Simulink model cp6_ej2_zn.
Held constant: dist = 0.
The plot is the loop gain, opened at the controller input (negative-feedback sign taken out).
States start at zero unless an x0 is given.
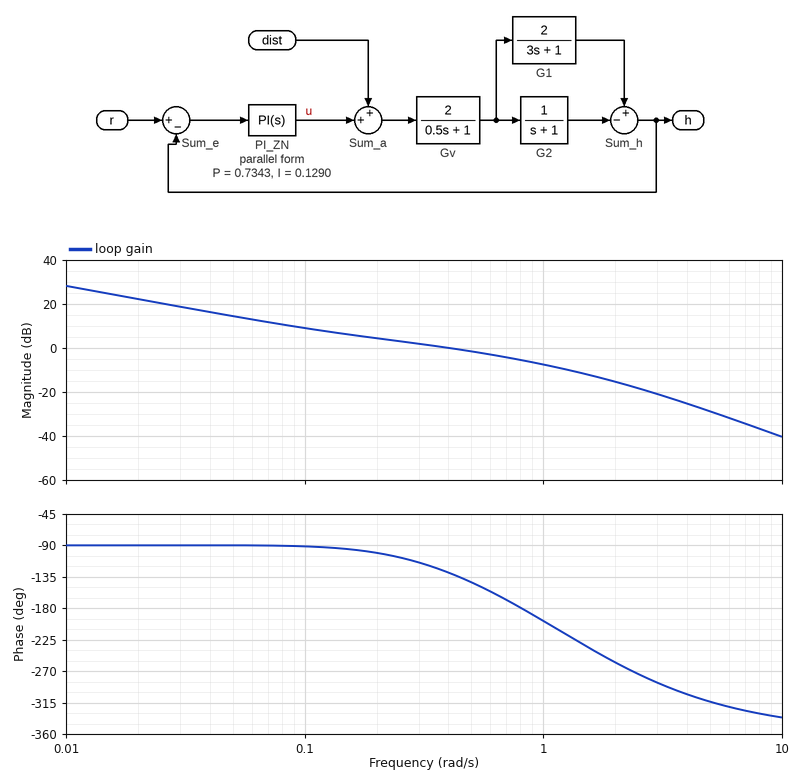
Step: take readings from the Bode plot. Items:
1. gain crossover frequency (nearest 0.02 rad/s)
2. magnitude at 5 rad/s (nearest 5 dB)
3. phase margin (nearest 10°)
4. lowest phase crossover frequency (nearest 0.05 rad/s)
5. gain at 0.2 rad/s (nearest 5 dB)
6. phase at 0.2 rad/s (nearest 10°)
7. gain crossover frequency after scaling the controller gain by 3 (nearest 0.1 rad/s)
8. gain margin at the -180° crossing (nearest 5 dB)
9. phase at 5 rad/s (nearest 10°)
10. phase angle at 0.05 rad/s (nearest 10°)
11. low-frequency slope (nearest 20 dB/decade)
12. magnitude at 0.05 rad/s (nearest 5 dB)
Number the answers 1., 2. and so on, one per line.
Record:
1. 0.40 rad/s
2. -30 dB
3. 50°
4. 0.80 rad/s
5. 5 dB
6. -100°
7. 1.2 rad/s
8. 5 dB
9. -310°
10. -90°
11. -20 dB/decade
12. 15 dB
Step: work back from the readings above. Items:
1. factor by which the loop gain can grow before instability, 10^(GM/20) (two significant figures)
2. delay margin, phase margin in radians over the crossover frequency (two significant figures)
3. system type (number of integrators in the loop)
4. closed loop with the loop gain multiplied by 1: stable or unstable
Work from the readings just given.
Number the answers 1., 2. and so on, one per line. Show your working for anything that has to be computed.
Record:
1. 10^(5 / 20) = 1.8
2. 50 × π / 180 / 0.4 = 2.2 s
3. 1
4. stable
